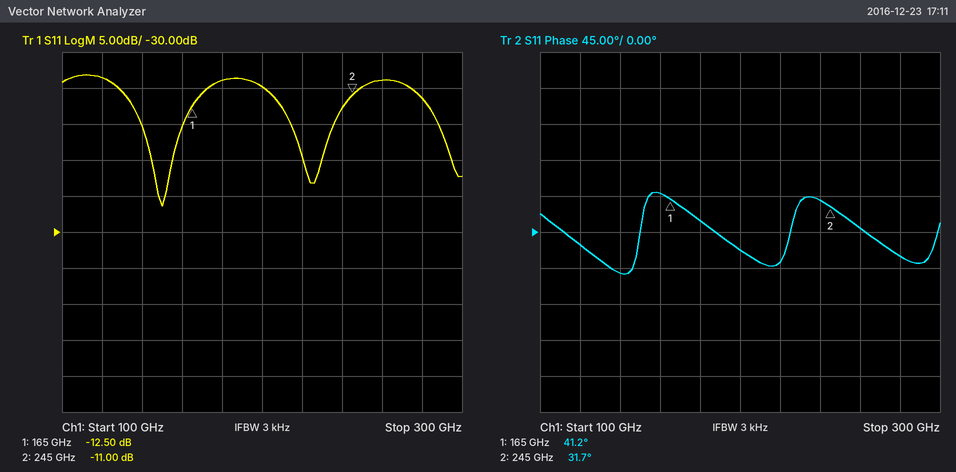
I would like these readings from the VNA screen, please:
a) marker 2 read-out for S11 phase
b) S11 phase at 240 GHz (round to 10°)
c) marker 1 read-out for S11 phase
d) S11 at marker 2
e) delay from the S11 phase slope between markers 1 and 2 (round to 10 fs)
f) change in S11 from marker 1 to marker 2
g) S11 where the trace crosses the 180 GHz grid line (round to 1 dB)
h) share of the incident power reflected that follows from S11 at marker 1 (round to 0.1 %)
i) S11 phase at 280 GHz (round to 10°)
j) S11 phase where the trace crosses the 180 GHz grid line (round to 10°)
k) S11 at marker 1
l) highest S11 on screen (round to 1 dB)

31.7°
40°
41.2°
-11.00 dB
330 fs
1.50 dB
-9 dB
5.6 %
-30°
10°
-12.50 dB
-8 dB
